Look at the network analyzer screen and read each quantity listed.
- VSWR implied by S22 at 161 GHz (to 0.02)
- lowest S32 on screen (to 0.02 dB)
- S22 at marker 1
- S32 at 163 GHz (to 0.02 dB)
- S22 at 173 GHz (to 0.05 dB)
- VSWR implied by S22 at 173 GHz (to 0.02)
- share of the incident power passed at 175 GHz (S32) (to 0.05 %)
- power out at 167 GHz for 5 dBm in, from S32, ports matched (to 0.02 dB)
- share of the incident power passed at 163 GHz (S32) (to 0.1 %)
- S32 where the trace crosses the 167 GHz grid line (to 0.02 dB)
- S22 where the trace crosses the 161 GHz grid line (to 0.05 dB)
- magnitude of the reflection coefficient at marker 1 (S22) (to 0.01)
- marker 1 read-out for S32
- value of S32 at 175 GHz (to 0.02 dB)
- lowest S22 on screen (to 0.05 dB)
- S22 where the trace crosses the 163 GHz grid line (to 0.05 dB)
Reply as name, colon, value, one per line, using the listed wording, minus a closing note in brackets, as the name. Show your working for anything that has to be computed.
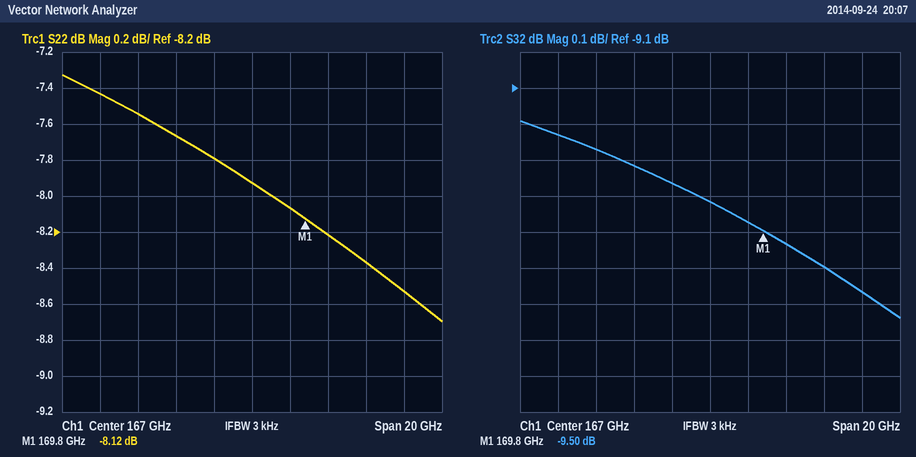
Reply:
VSWR implied by S22 at 161 GHz: |Γ| = 10^(-7.55/20) = 0.4193; VSWR = (1 + 0.4193)/(1 − 0.4193) ≈ 2.44
lowest S32 on screen: -9.74 dB
S22 at marker 1: -8.12 dB
S32 at 163 GHz: -9.32 dB
S22 at 173 GHz: -8.35 dB
VSWR implied by S22 at 173 GHz: |Γ| = 10^(-8.35/20) = 0.3824; VSWR = (1 + 0.3824)/(1 − 0.3824) ≈ 2.24
share of the incident power passed at 175 GHz (S32): 10^(-9.66/10) ≈ 10.80 %
power out at 167 GHz for 5 dBm in, from S32, ports matched: 5 dBm + (-9.42 dB) = -4.42 dBm
share of the incident power passed at 163 GHz (S32): 10^(-9.32/10) ≈ 11.7 %
S32 where the trace crosses the 167 GHz grid line: -9.42 dB
S22 where the trace crosses the 161 GHz grid line: -7.55 dB
magnitude of the reflection coefficient at marker 1 (S22): 10^(-8.12/20) ≈ 0.39
marker 1 read-out for S32: -9.50 dB
value of S32 at 175 GHz: -9.66 dB
lowest S22 on screen: -8.70 dB
S22 where the trace crosses the 163 GHz grid line: -7.65 dB
